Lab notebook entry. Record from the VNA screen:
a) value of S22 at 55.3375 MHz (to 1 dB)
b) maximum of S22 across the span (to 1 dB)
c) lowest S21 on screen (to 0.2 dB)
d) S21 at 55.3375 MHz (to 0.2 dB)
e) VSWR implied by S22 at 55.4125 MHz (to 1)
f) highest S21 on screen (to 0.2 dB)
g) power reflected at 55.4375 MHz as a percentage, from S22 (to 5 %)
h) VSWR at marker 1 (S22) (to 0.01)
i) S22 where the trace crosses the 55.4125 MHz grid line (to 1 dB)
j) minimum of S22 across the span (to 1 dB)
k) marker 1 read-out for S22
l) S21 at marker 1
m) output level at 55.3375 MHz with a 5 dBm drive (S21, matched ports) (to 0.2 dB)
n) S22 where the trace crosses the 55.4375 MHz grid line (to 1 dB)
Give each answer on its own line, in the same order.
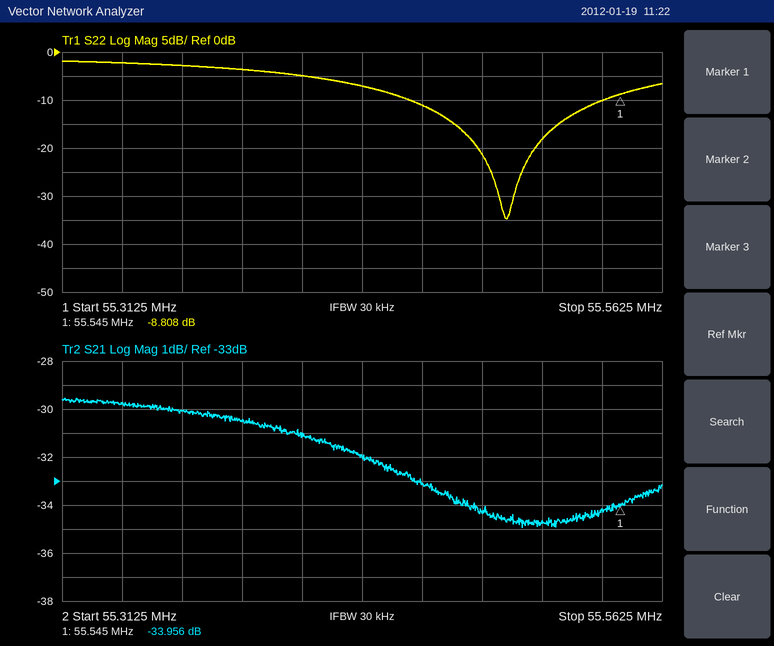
-2 dB
-2 dB
-35.0 dB
-29.8 dB
4
-29.6 dB
20 %
2.14
-5 dB
-35 dB
-8.808 dB
-33.956 dB
-24.8 dBm
-7 dB
